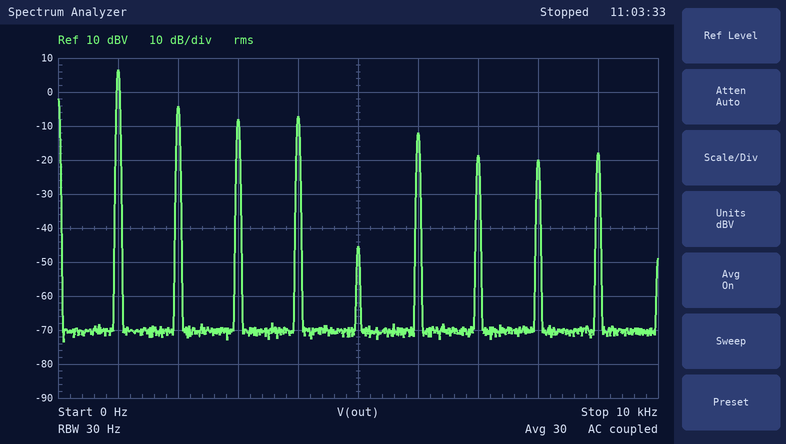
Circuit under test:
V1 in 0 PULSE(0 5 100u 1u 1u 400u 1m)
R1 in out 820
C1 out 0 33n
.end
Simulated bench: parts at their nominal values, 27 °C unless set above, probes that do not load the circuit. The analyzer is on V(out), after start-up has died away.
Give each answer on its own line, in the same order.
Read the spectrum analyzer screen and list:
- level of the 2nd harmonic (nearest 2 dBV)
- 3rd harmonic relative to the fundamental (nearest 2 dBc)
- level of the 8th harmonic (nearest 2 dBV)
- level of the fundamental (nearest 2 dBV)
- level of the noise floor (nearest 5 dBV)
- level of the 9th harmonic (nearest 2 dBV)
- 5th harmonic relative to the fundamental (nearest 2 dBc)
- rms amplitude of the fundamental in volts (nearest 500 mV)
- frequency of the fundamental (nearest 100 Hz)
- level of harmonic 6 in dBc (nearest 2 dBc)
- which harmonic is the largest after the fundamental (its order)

-4 dBV
-14 dBc
-20 dBV
6 dBV
-70 dBV
-18 dBV
-52 dBc
2.0 V
1.0 kHz
-18 dBc
2
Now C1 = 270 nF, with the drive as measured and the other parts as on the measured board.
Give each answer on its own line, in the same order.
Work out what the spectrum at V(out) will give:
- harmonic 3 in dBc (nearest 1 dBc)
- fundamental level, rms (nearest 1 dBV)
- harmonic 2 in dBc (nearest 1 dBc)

-22 dBc
2 dBV
-15 dBc
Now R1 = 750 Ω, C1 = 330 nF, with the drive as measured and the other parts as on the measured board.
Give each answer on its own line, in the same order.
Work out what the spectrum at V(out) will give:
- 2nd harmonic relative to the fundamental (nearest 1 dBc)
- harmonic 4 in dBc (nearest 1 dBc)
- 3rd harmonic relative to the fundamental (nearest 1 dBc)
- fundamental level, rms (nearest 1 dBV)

-15 dBc
-23 dBc
-22 dBc
1 dBV
